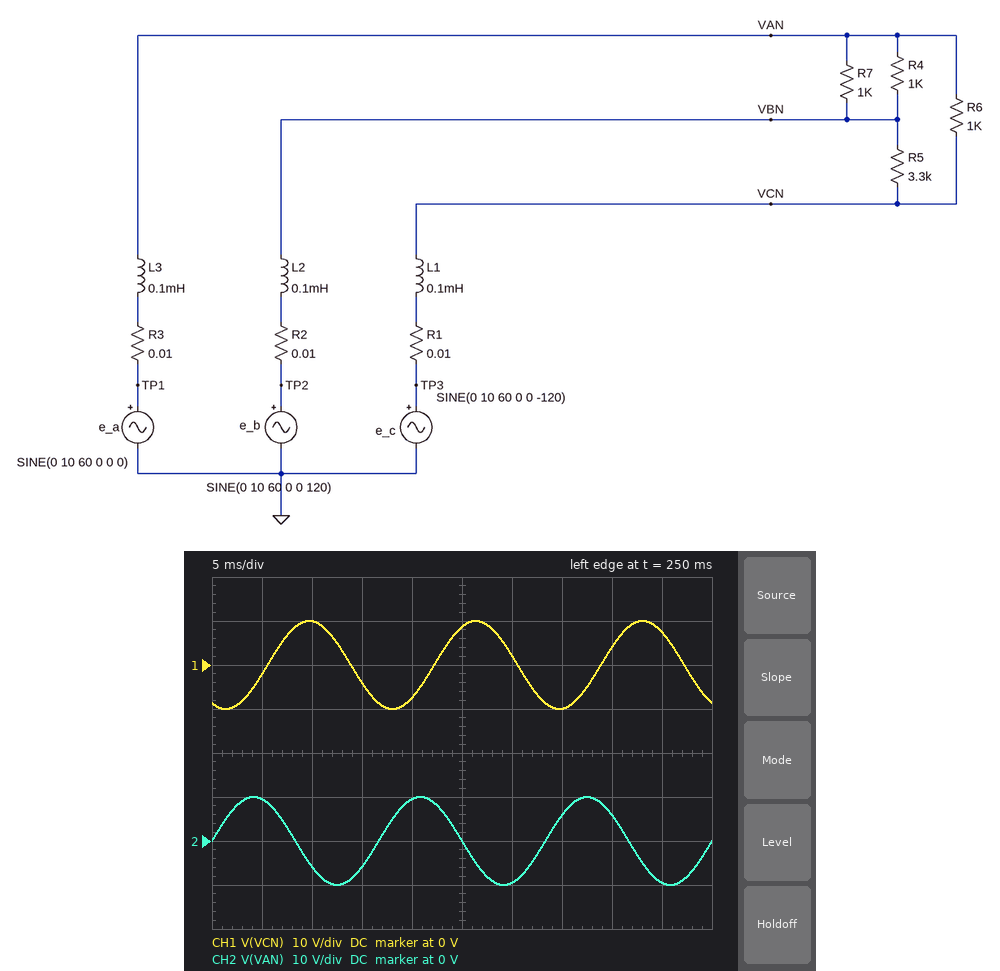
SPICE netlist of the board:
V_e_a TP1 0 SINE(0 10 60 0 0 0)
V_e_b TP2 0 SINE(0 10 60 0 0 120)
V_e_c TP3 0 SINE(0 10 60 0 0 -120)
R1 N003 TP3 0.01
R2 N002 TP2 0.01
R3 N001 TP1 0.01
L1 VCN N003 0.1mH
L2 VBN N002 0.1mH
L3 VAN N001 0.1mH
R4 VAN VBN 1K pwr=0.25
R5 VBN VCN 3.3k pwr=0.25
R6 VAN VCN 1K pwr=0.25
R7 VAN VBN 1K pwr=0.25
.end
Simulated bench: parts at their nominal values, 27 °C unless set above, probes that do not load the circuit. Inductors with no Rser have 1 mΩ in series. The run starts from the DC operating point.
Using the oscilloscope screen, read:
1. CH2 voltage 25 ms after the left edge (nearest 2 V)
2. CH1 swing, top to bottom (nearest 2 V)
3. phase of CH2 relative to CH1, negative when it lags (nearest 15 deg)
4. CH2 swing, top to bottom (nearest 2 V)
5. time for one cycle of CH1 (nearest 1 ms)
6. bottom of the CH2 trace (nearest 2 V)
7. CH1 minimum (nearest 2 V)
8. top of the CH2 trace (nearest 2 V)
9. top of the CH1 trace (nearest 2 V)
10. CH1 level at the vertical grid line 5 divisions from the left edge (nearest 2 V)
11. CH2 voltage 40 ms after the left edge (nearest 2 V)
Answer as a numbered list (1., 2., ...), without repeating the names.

1. 0 V
2. 20 V
3. 120 deg
4. 20 V
5. 17 ms
6. -10 V
7. -10 V
8. 10 V
9. 10 V
10. 8 V
11. 6 V
